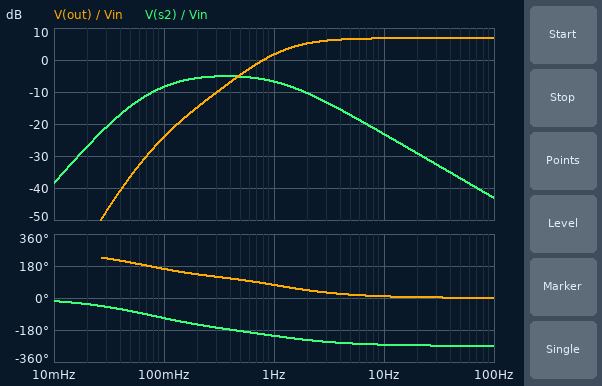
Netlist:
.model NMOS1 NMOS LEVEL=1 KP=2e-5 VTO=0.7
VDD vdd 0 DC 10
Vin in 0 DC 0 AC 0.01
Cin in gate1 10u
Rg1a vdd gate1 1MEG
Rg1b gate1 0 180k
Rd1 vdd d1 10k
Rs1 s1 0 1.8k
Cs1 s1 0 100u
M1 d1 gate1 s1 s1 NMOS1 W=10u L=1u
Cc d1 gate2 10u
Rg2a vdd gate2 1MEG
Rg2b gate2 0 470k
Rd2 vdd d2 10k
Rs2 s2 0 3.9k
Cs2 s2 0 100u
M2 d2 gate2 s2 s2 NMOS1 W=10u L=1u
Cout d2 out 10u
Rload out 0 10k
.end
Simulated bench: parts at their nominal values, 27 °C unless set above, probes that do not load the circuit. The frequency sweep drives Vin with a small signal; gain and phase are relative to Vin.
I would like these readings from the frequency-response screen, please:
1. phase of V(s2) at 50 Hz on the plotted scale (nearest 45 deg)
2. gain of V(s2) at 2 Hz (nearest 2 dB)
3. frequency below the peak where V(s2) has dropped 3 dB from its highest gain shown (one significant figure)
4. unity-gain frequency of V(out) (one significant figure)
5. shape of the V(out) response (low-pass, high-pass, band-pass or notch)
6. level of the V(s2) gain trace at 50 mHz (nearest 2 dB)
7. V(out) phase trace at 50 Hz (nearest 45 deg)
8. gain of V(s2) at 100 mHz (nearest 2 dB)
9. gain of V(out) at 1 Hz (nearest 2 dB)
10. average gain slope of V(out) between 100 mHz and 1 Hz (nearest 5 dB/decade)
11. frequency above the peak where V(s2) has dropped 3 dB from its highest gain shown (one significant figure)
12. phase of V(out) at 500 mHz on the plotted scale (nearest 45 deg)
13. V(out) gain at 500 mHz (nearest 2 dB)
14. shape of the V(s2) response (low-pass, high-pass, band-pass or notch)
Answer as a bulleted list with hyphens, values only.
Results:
- -270 deg
- -10 dB
- 100 mHz
- 800 mHz
- high-pass
- -14 dB
- 0 deg
- -8 dB
- 2 dB
- 25 dB/decade
- 1 Hz
- 90 deg
- -4 dB
- band-pass
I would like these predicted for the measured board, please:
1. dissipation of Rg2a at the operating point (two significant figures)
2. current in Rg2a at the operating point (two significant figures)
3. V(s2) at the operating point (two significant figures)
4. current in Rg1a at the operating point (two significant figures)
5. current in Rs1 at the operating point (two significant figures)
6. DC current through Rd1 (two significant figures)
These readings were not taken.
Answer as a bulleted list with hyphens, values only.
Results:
- 46 µW
- 6.8 µA
- 940 mV
- 8.5 µA
- 53 µA
- 53 µA
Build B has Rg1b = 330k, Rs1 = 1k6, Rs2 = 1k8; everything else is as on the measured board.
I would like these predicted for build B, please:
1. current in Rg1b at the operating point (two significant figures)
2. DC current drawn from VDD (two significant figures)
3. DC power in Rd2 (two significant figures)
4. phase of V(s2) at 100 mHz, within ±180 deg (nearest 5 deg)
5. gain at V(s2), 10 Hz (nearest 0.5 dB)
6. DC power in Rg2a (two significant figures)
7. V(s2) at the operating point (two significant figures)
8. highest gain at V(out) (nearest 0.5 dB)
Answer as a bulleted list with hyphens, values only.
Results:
- 7.5 µA
- 570 µA
- 1.2 mW
- -125 deg
- -15.5 dB
- 46 µW
- 630 mV
- 14.5 dB
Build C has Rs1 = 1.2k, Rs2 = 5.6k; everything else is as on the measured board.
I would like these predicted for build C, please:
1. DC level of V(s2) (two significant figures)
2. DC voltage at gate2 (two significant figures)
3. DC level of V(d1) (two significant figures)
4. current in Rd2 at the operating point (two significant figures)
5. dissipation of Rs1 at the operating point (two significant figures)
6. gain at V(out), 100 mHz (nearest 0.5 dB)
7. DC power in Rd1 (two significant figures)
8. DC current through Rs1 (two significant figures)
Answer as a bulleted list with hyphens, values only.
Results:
- 1.1 V
- 3.2 V
- 9.4 V
- 200 µA
- 3.9 µW
- -25.0 dB
- 33 µW
- 57 µA
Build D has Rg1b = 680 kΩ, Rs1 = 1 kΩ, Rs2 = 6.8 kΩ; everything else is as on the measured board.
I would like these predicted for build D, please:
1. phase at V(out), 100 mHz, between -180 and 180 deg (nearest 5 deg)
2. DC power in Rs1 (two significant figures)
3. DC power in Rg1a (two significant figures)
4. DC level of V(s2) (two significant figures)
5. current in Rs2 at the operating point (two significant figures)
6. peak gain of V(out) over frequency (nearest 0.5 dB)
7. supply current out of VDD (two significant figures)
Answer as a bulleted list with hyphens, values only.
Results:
- 145 deg
- 480 µW
- 35 µW
- 1.2 V
- 170 µA
- 11.5 dB
- 880 µA
